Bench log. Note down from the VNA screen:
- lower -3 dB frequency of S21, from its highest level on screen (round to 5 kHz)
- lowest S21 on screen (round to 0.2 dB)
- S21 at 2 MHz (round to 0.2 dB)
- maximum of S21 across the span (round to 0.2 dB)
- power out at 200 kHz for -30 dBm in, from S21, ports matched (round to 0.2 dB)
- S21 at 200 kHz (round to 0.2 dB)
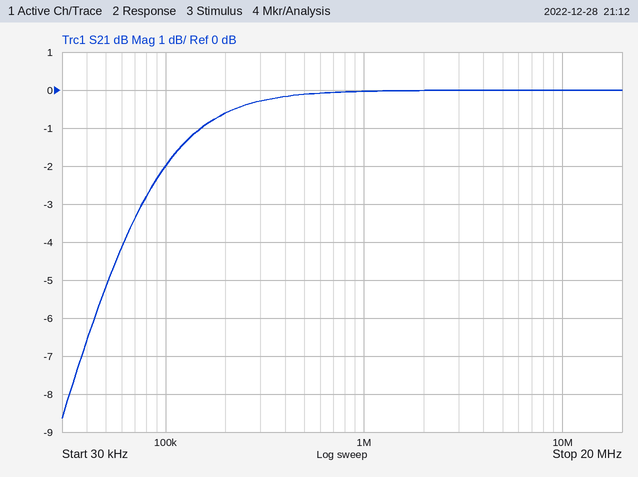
75 kHz
-8.6 dB
0.0 dB
0.0 dB
-30.6 dBm
-0.6 dB
